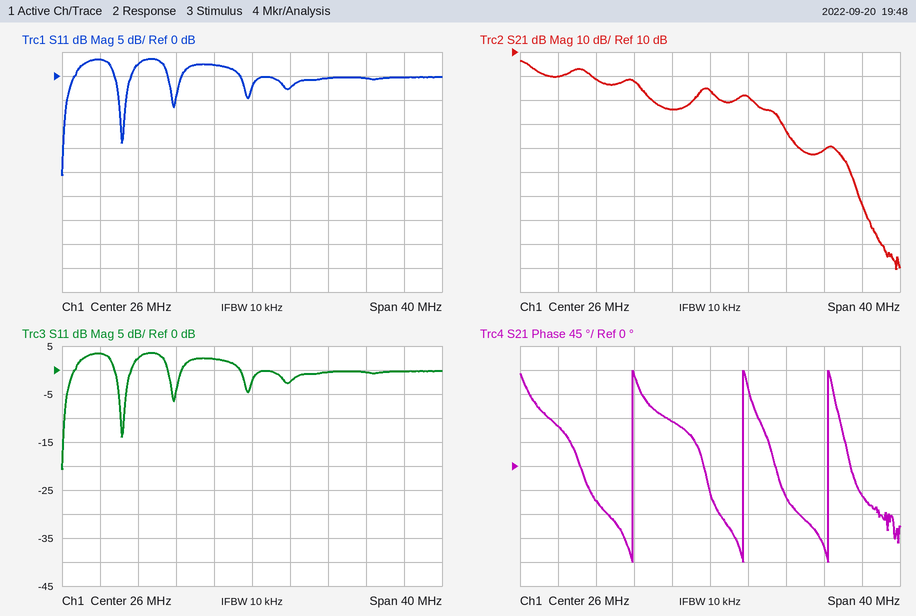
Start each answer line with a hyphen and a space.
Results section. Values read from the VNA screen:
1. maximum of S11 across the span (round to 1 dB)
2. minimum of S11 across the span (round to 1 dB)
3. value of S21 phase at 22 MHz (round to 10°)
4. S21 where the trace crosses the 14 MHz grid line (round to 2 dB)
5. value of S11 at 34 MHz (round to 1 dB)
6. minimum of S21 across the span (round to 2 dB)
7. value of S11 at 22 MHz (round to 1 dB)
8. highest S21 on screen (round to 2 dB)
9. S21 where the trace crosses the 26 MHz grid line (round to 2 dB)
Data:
- 4 dB
- -21 dB
- 80°
- -2 dB
- 0 dB
- -80 dB
- 2 dB
- 6 dB
- -6 dB
